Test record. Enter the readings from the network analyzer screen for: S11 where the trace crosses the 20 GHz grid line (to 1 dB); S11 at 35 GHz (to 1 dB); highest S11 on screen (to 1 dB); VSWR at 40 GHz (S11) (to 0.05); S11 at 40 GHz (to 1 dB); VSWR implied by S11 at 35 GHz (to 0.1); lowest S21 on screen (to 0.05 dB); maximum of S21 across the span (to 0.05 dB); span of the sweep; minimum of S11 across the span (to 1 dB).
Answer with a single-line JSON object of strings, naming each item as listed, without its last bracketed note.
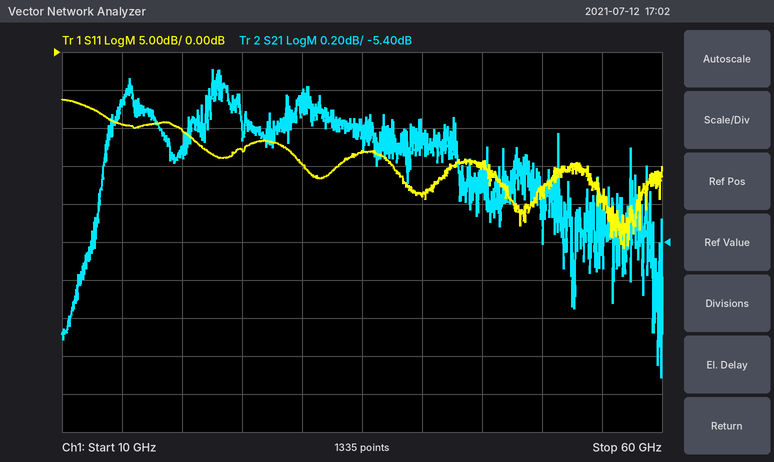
{"S11 where the trace crosses the 20 GHz grid line": "-10 dB", "S11 at 35 GHz": "-13 dB", "highest S11 on screen": "-6 dB", "VSWR at 40 GHz (S11)": "1.25", "S11 at 40 GHz": "-19 dB", "VSWR implied by S11 at 35 GHz": "1.6", "lowest S21 on screen": "-6.10 dB", "maximum of S21 across the span": "-4.50 dB", "span of the sweep": "50 GHz", "minimum of S11 across the span": "-26 dB"}
